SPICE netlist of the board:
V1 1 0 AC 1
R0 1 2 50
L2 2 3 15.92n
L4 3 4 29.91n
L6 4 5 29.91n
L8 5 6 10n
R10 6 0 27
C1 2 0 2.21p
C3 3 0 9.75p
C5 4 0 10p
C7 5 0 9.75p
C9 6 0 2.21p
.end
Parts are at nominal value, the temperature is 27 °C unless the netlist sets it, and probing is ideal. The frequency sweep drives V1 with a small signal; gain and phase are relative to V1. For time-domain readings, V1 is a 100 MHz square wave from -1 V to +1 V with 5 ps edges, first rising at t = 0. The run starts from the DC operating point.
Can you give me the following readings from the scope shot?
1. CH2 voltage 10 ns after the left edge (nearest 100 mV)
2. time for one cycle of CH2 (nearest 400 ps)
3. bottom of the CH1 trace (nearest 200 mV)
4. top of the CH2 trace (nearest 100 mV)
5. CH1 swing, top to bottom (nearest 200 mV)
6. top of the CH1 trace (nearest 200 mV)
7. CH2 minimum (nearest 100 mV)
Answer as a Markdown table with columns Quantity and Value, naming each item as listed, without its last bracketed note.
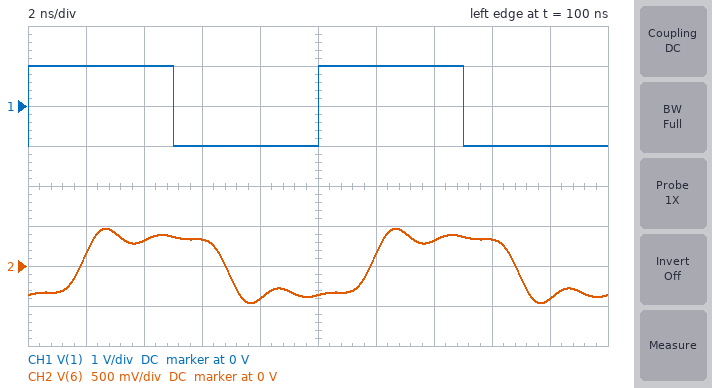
| Quantity | Value |
|---|---|
| CH2 voltage 10 ns after the left edge | -400 mV |
| time for one cycle of CH2 | 10.0 ns |
| bottom of the CH1 trace | -1.0 V |
| top of the CH2 trace | 500 mV |
| CH1 swing, top to bottom | 2.0 V |
| top of the CH1 trace | 1.0 V |
| CH2 minimum | -500 mV |
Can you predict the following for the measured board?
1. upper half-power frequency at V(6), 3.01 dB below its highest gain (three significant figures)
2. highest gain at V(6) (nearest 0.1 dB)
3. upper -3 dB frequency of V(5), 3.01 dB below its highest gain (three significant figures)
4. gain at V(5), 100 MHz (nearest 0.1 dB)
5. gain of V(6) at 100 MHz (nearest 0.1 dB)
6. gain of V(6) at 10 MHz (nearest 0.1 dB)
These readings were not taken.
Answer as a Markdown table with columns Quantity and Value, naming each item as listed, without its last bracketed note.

| Quantity | Value |
|---|---|
| upper half-power frequency at V(6), 3.01 dB below its highest gain | 541 MHz |
| highest gain at V(6) | -8.8 dB |
| upper -3 dB frequency of V(5), 3.01 dB below its highest gain | 554 MHz |
| gain at V(5), 100 MHz | -9.0 dB |
| gain of V(6) at 100 MHz | -9.2 dB |
| gain of V(6) at 10 MHz | -9.1 dB |
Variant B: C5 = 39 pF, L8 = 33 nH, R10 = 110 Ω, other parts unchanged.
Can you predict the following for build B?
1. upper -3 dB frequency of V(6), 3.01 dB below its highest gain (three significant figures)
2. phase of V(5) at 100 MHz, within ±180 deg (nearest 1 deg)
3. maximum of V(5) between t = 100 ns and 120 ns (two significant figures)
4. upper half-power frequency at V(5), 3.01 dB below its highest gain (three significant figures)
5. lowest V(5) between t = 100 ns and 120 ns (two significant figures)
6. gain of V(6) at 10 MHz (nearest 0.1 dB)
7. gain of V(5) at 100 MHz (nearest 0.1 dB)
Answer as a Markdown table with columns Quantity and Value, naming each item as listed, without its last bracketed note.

| Quantity | Value |
|---|---|
| upper -3 dB frequency of V(6), 3.01 dB below its highest gain | 164 MHz |
| phase of V(5) at 100 MHz, within ±180 deg | -83 deg |
| maximum of V(5) between t = 100 ns and 120 ns | 660 mV |
| upper half-power frequency at V(5), 3.01 dB below its highest gain | 149 MHz |
| lowest V(5) between t = 100 ns and 120 ns | -660 mV |
| gain of V(6) at 10 MHz | -3.3 dB |
| gain of V(5) at 100 MHz | -5.2 dB |
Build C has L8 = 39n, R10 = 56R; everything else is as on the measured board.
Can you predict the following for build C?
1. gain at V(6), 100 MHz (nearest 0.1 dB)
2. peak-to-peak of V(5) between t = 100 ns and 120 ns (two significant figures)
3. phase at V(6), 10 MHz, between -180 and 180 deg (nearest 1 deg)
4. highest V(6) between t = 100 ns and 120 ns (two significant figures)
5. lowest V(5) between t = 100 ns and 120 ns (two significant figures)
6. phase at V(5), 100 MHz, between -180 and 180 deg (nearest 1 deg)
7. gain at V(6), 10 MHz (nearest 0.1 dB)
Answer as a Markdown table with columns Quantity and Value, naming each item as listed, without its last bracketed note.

| Quantity | Value |
|---|---|
| gain at V(6), 100 MHz | -5.6 dB |
| peak-to-peak of V(5) between t = 100 ns and 120 ns | 2.1 V |
| phase at V(6), 10 MHz, between -180 and 180 deg | -7 deg |
| highest V(6) between t = 100 ns and 120 ns | 710 mV |
| lowest V(5) between t = 100 ns and 120 ns | -1.0 V |
| phase at V(5), 100 MHz, between -180 and 180 deg | -47 deg |
| gain at V(6), 10 MHz | -5.5 dB |
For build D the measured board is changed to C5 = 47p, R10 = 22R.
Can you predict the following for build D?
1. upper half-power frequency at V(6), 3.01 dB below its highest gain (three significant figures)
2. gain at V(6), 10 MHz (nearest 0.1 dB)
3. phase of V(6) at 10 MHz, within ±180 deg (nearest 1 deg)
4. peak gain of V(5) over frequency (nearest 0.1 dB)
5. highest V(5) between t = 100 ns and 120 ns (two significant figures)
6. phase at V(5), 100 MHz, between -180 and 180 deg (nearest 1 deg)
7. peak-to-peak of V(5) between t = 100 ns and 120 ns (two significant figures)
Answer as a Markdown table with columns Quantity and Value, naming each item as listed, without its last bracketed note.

| Quantity | Value |
|---|---|
| upper half-power frequency at V(6), 3.01 dB below its highest gain | 184 MHz |
| gain at V(6), 10 MHz | -10.3 dB |
| phase of V(6) at 10 MHz, within ±180 deg | -8 deg |
| peak gain of V(5) over frequency | -9.4 dB |
| highest V(5) between t = 100 ns and 120 ns | 390 mV |
| phase at V(5), 100 MHz, between -180 and 180 deg | -75 deg |
| peak-to-peak of V(5) between t = 100 ns and 120 ns | 780 mV |
